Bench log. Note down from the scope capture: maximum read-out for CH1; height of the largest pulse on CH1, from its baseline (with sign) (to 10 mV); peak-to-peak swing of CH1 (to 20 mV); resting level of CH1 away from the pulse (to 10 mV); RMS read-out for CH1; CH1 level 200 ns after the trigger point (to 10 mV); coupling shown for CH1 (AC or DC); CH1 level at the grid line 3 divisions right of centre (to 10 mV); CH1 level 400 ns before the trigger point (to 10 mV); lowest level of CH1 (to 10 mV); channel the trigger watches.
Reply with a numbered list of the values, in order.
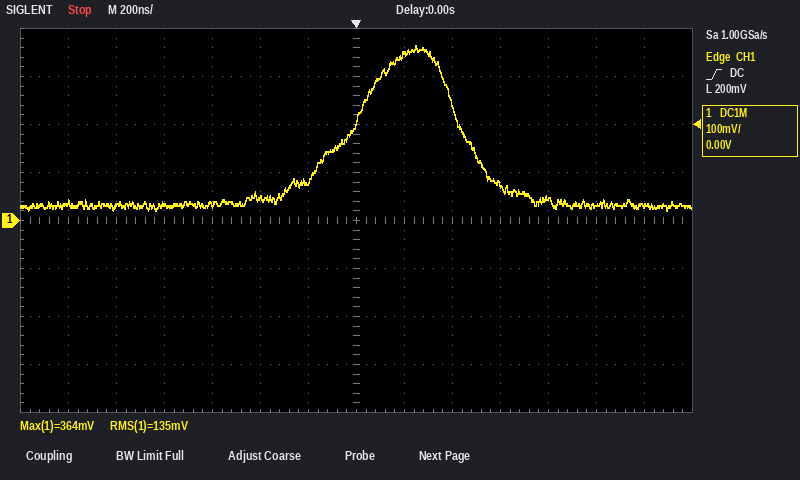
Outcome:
1. 364 mV
2. +330 mV
3. 340 mV
4. 30 mV
5. 135 mV
6. 350 mV
7. DC
8. 80 mV
9. 50 mV
10. 20 mV
11. CH1
